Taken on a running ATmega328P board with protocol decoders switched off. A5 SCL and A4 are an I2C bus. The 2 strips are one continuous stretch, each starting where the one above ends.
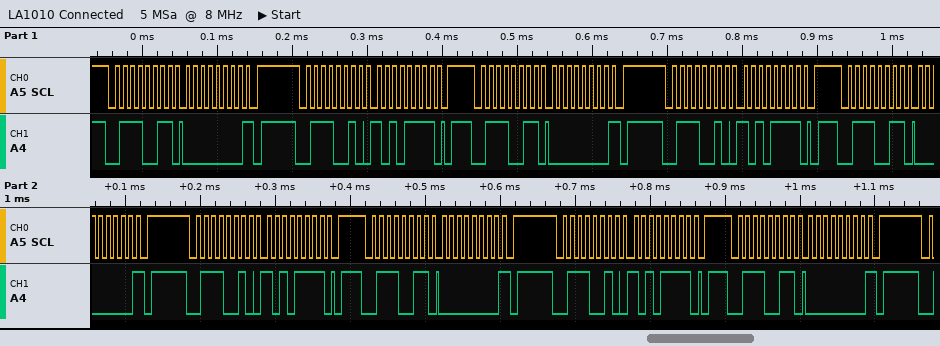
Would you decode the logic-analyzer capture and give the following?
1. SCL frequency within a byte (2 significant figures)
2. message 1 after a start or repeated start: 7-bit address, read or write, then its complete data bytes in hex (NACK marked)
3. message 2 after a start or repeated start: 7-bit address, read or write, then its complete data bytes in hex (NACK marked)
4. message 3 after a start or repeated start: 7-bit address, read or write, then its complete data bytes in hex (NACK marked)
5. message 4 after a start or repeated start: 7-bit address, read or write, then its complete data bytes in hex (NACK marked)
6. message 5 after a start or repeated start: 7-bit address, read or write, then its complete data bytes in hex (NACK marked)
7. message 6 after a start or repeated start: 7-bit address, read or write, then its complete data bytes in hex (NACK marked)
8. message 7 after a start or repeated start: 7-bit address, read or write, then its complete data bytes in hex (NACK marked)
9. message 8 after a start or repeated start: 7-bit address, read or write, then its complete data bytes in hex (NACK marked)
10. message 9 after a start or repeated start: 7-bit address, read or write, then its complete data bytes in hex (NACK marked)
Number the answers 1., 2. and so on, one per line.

1. 100 kHz
2. 0x39 read: 00 NACK
3. 0x39 write: AF
4. 0x39 read: 00 NACK
5. 0x39 write: AF
6. 0x39 read: 00 NACK
7. 0x39 write: AF
8. 0x39 read: 00 NACK
9. 0x39 write: AF
10. 0x39 read: 00 NACK
